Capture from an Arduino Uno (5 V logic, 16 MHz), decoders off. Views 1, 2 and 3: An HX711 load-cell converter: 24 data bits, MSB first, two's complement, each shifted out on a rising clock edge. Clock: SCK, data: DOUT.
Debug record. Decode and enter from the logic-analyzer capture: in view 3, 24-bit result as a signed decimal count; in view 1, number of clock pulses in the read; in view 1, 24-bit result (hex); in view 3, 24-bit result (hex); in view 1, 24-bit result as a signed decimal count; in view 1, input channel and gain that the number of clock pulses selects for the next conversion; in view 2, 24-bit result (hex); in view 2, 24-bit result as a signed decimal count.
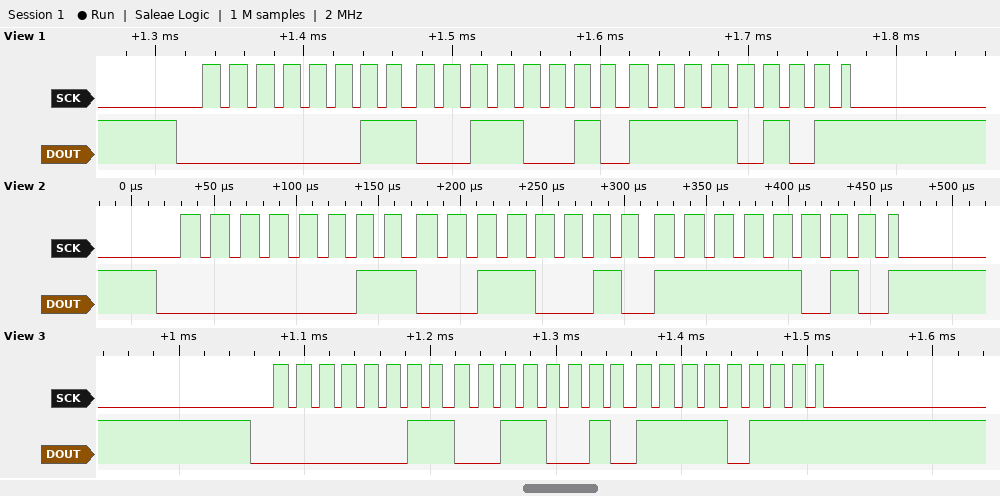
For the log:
209655
25
0x0332F5
0x0332F7
209653
channel A, gain 128
0x0332FA
209658
